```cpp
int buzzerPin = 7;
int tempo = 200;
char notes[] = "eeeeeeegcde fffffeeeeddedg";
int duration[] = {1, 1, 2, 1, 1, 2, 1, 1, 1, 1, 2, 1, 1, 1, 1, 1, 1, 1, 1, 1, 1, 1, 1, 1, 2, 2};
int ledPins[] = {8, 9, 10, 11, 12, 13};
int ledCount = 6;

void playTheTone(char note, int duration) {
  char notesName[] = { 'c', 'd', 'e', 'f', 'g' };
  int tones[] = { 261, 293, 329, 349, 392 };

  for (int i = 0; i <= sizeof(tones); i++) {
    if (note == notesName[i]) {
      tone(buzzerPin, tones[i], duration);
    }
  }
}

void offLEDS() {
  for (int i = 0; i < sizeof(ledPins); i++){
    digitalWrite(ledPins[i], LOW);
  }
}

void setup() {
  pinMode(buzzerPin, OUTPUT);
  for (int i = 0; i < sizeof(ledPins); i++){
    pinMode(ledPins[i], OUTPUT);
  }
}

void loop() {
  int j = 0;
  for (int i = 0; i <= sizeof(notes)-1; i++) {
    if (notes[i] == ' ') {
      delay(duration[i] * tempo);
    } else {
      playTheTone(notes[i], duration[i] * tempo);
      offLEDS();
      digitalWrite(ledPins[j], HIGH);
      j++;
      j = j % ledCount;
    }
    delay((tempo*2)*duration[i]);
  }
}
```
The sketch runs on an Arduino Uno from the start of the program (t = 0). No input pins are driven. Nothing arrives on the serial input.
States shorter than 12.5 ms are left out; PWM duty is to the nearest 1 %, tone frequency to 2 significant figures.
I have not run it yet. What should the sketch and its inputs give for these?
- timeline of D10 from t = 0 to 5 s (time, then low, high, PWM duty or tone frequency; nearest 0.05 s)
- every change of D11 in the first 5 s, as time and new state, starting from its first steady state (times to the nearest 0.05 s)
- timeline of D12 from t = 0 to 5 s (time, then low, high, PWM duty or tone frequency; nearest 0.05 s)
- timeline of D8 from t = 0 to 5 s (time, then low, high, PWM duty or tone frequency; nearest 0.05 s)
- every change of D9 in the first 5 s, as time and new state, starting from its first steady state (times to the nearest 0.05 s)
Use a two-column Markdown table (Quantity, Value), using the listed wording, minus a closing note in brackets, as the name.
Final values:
| Quantity | Value |
|---|---|
| timeline of D10 from t = 0 to 5 s | 0 s low; 0.8 s high; 1.6 s low; 4 s high; 4.4 s low |
| every change of D11 in the first 5 s, as time and new state, starting from its first steady state | 0 s low; 1.6 s high; 2 s low; 4.4 s high; 4.8 s low |
| timeline of D12 from t = 0 to 5 s | 0 s low; 2 s high; 2.4 s low; 4.8 s high |
| timeline of D8 from t = 0 to 5 s | 0 s high; 0.4 s low; 3.2 s high; 3.6 s low |
| every change of D9 in the first 5 s, as time and new state, starting from its first steady state | 0 s low; 0.4 s high; 0.8 s low; 3.6 s high; 4 s low |
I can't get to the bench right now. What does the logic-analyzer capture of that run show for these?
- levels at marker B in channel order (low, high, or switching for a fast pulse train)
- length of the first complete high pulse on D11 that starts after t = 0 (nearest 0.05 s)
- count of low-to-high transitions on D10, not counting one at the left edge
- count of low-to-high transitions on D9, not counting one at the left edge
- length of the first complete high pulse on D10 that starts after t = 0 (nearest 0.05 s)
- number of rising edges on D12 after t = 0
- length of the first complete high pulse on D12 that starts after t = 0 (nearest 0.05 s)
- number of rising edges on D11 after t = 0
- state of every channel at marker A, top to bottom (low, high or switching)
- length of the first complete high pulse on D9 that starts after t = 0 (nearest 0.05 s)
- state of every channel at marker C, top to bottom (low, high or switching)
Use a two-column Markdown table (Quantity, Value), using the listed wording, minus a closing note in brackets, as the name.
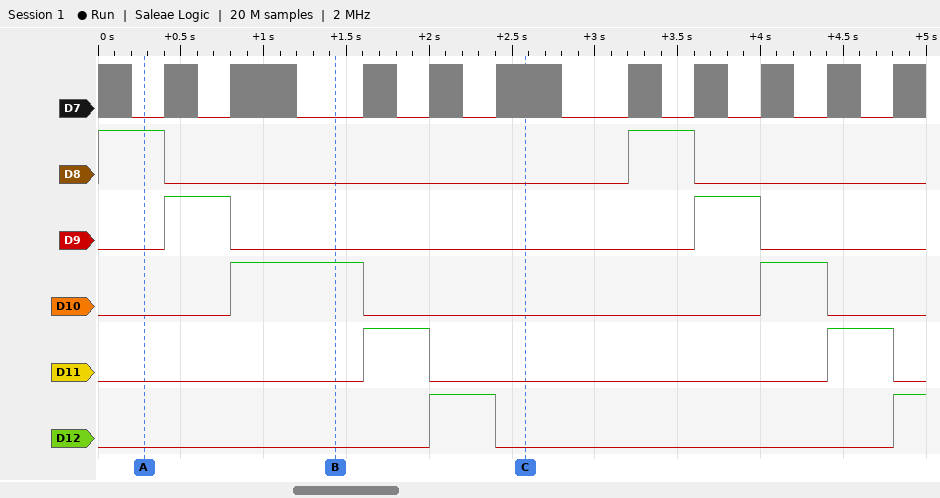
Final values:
| Quantity | Value |
|---|---|
| levels at marker B in channel order | D7 low, D8 low, D9 low, D10 high, D11 low, D12 low |
| length of the first complete high pulse on D11 that starts after t = 0 | 0.40 s |
| count of low-to-high transitions on D10, not counting one at the left edge | 2 |
| count of low-to-high transitions on D9, not counting one at the left edge | 2 |
| length of the first complete high pulse on D10 that starts after t = 0 | 0.80 s |
| number of rising edges on D12 after t = 0 | 2 |
| length of the first complete high pulse on D12 that starts after t = 0 | 0.40 s |
| number of rising edges on D11 after t = 0 | 2 |
| state of every channel at marker A, top to bottom | D7 low, D8 high, D9 low, D10 low, D11 low, D12 low |
| length of the first complete high pulse on D9 that starts after t = 0 | 0.40 s |
| state of every channel at marker C, top to bottom | D7 switching, D8 low, D9 low, D10 low, D11 low, D12 low |
